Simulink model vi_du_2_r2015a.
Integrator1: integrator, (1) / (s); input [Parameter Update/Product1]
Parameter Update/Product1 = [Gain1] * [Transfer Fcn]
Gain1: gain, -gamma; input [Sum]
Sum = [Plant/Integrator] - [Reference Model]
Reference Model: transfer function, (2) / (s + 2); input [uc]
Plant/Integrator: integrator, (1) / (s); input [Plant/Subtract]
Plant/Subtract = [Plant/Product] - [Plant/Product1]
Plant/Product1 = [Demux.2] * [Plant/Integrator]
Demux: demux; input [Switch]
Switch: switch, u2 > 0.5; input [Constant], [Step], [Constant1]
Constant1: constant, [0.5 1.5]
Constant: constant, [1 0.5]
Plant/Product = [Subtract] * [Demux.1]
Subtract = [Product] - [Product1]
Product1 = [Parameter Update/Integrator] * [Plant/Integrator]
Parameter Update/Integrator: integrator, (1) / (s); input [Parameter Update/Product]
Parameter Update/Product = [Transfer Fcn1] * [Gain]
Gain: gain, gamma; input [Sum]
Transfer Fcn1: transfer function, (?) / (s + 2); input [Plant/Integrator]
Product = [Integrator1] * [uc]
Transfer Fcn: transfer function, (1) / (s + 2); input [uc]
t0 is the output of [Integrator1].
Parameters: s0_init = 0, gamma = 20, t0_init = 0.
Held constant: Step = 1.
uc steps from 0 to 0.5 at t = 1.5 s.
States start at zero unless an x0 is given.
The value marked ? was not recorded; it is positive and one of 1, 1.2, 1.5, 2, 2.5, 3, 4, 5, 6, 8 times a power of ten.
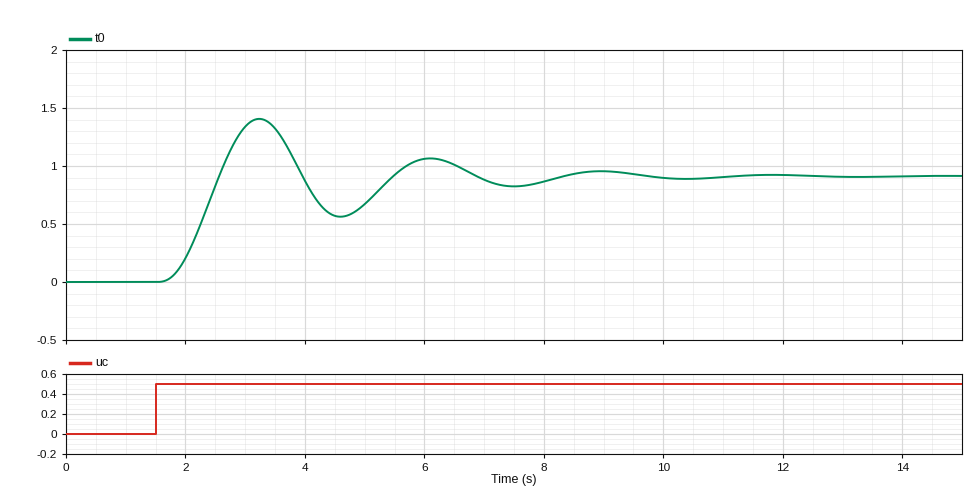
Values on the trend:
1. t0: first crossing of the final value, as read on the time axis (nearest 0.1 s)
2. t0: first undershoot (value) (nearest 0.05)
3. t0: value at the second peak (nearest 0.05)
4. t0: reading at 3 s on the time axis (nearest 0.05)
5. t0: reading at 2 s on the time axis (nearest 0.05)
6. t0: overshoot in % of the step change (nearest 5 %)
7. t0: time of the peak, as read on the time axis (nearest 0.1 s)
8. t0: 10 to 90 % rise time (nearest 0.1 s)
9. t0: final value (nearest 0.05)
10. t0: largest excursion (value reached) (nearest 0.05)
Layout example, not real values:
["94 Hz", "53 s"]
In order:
["2.6 s", "0.55", "1.05", "1.35", "0.20", "55 %", "3.2 s", "0.6 s", "0.90", "1.40"]
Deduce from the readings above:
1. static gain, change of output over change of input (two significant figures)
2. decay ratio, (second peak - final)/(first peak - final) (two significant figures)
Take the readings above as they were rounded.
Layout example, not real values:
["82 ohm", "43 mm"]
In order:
["1.8", "0.30"]
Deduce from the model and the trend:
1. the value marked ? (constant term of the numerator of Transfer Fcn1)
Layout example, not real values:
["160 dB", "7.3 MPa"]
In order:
["1"]
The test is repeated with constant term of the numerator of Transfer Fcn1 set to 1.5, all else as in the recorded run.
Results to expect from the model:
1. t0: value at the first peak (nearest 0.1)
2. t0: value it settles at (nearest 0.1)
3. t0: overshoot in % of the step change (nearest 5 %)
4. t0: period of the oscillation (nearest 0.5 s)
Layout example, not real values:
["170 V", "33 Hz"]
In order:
["1.4", "1.0", "45 %", "2.5 s"]
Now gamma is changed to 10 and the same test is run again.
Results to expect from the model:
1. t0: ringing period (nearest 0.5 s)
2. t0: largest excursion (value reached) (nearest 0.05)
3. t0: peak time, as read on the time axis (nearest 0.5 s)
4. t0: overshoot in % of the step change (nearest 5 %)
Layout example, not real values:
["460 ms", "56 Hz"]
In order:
["4.0 s", "1.10", "4.0 s", "40 %"]
